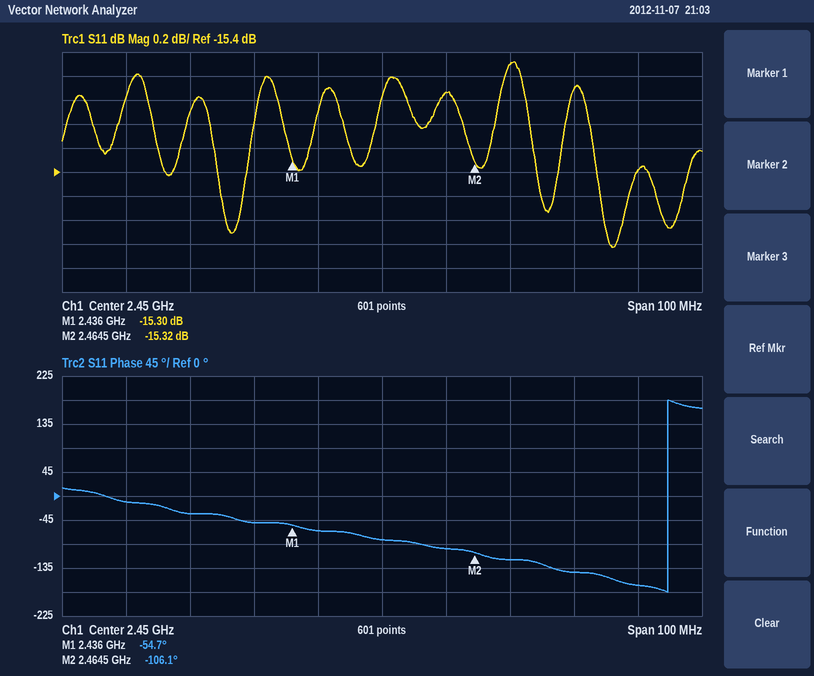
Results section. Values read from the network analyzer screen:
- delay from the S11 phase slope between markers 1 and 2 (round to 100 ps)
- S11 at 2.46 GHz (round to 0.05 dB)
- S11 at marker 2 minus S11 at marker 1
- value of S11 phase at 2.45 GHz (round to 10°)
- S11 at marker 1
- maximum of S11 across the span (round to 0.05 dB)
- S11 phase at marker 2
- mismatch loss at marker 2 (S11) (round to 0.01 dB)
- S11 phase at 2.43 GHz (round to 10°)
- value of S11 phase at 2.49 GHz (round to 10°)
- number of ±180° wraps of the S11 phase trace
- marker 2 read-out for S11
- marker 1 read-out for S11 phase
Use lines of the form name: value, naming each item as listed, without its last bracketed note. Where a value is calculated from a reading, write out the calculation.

delay from the S11 phase slope between markers 1 and 2: −(-106.1° − (-54.7°))/(360° × 28.5 MHz) ≈ 5.0 ns
S11 at 2.46 GHz: -14.75 dB
S11 at marker 2 minus S11 at marker 1: -15.32 − (-15.3) = -0.02 dB
value of S11 phase at 2.45 GHz: -80°
S11 at marker 1: -15.30 dB
maximum of S11 across the span: -14.50 dB
S11 phase at marker 2: -106.1°
mismatch loss at marker 2 (S11): −10 log10(1 − 10^(-15.32/10)) ≈ 0.13 dB
S11 phase at 2.43 GHz: -50°
value of S11 phase at 2.49 GHz: -170°
number of ±180° wraps of the S11 phase trace: 1
marker 2 read-out for S11: -15.32 dB
marker 1 read-out for S11 phase: -54.7°
